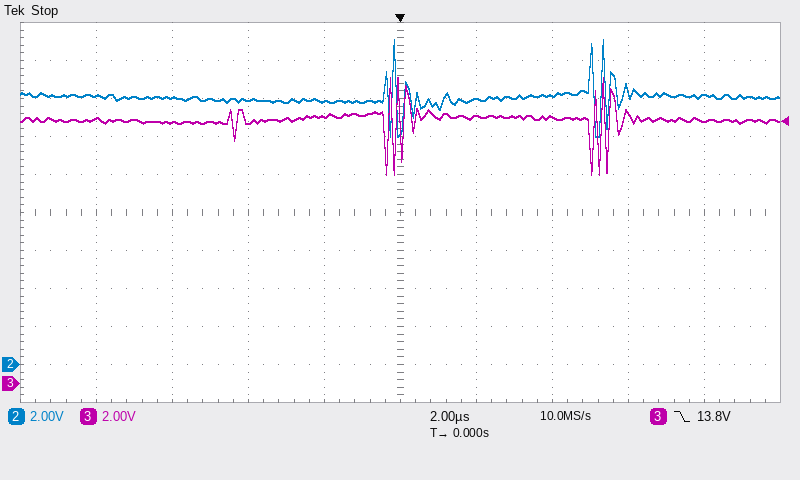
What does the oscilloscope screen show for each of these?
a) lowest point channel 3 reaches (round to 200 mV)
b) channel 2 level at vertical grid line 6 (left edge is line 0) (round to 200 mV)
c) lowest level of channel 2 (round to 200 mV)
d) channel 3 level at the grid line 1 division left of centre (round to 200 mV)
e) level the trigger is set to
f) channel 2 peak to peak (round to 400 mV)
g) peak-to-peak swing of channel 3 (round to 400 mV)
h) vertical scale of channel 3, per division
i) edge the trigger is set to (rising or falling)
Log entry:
11.0 V
14.0 V
12.0 V
14.0 V
13.8 V
5.2 V
5.2 V
2 V
falling
